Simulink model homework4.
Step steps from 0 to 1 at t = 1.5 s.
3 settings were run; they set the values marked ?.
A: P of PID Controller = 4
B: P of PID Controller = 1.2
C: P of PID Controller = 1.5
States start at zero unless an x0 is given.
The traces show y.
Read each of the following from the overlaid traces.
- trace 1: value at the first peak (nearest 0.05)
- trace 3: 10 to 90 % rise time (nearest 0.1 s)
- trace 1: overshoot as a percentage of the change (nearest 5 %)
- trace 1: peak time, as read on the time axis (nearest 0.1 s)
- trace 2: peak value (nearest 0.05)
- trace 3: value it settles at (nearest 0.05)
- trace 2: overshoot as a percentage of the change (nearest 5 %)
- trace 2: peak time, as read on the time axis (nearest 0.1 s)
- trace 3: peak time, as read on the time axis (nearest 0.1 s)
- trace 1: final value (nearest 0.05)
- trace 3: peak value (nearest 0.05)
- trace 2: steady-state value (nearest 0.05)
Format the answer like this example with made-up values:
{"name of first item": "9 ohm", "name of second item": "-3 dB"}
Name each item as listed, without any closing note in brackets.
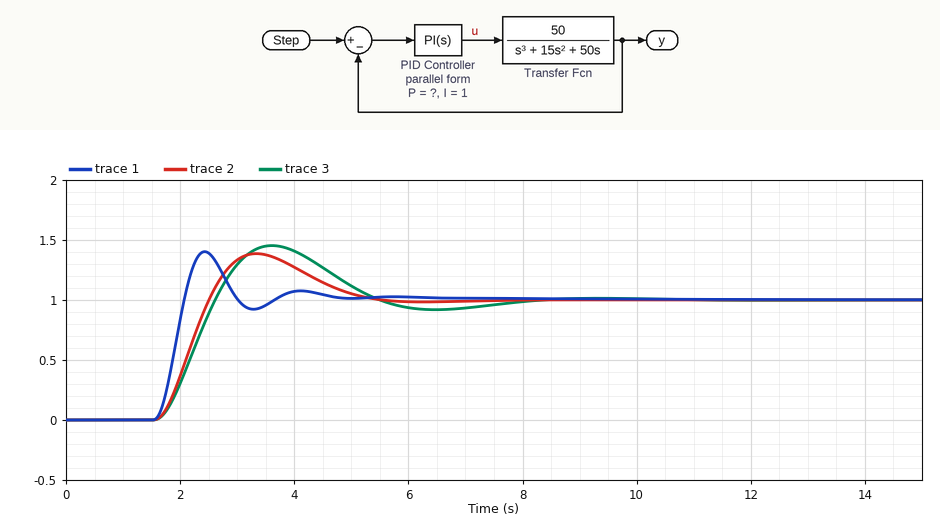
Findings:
{"trace 1: value at the first peak": "1.40", "trace 3: 10 to 90 % rise time": "0.7 s", "trace 1: overshoot as a percentage of the change": "40 %", "trace 1: peak time, as read on the time axis": "2.4 s", "trace 2: peak value": "1.40", "trace 3: value it settles at": "1.00", "trace 2: overshoot as a percentage of the change": "40 %", "trace 2: peak time, as read on the time axis": "3.3 s", "trace 3: peak time, as read on the time axis": "3.6 s", "trace 1: final value": "1.00", "trace 3: peak value": "1.45", "trace 2: steady-state value": "1.00"}
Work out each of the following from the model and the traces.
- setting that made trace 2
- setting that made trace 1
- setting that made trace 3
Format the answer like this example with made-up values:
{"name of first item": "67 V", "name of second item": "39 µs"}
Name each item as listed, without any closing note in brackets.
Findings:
{"setting that made trace 2": "C", "setting that made trace 1": "A", "setting that made trace 3": "B"}
